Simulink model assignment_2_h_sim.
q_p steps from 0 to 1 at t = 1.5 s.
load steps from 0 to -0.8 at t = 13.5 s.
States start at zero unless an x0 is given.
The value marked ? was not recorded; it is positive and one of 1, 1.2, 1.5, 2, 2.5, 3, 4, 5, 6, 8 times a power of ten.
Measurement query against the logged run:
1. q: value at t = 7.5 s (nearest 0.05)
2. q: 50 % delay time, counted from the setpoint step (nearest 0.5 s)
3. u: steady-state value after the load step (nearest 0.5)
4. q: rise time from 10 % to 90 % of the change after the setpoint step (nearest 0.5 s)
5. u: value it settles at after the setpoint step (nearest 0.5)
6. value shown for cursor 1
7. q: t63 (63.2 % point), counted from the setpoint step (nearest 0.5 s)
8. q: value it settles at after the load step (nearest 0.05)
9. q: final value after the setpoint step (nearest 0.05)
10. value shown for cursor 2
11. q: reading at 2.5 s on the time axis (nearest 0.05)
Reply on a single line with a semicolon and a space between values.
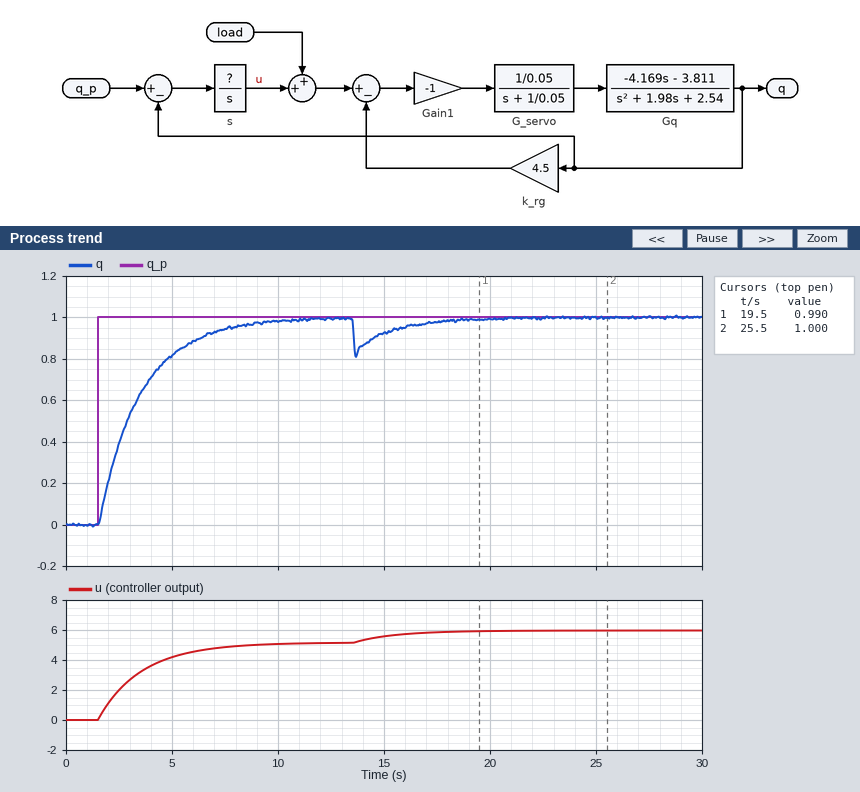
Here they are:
0.95; 1.5 s; 6.0; 4.5 s; 5.0; 0.990; 2.0 s; 1.00; 1.00; 1.000; 0.40
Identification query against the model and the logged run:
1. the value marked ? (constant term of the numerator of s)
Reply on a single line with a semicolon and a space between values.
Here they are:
2.5
